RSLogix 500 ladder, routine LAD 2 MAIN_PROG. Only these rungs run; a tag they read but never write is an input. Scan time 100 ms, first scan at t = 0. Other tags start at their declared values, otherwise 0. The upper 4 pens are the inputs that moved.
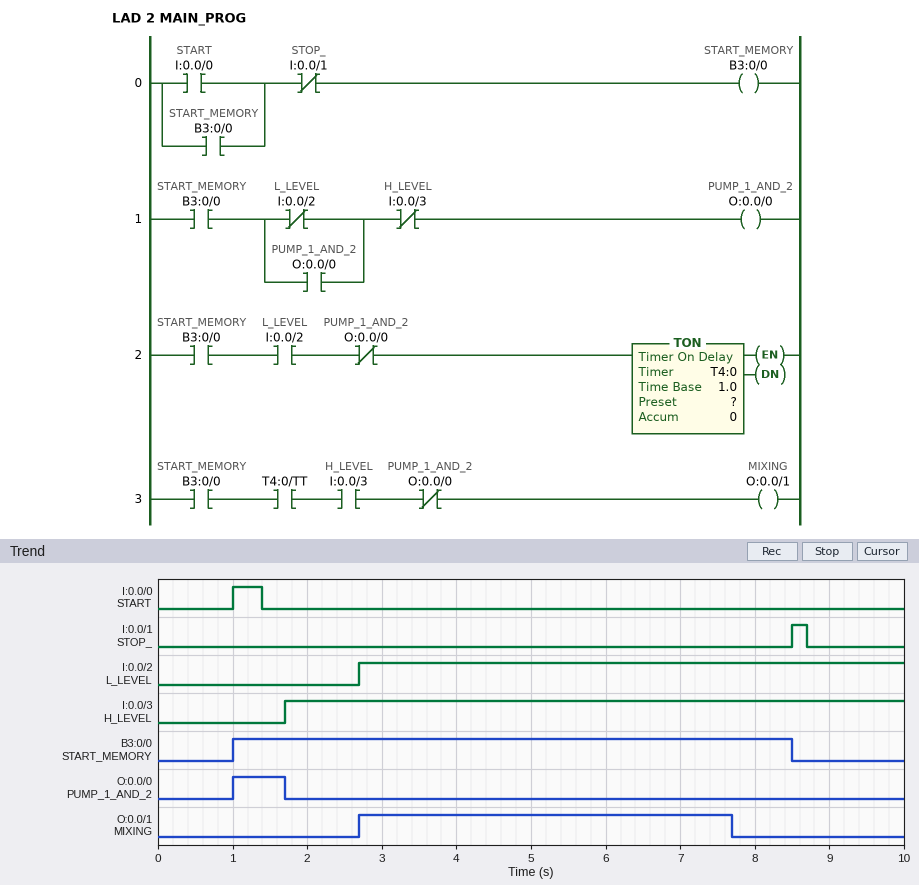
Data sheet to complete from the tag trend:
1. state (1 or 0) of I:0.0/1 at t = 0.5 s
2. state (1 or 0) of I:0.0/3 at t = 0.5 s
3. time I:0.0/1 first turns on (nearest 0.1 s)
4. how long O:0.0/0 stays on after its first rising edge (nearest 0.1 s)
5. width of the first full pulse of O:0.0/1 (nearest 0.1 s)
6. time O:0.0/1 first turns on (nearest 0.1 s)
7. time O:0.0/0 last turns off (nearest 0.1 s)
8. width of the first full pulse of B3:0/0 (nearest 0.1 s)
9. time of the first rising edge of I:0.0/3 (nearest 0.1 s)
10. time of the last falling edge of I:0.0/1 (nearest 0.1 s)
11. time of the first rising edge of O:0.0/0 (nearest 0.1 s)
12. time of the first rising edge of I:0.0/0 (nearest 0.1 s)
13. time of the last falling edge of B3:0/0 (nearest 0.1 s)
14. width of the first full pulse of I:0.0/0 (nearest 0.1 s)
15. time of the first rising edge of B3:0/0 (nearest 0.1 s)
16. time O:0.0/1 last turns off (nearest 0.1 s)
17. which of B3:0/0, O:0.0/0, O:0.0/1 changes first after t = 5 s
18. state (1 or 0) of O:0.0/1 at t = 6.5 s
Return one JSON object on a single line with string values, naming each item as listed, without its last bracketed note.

{"state (1 or 0) of I:0.0/1 at t = 0.5 s": "0", "state (1 or 0) of I:0.0/3 at t = 0.5 s": "0", "time I:0.0/1 first turns on": "8.5 s", "how long O:0.0/0 stays on after its first rising edge": "0.7 s", "width of the first full pulse of O:0.0/1": "5.0 s", "time O:0.0/1 first turns on": "2.7 s", "time O:0.0/0 last turns off": "1.7 s", "width of the first full pulse of B3:0/0": "7.5 s", "time of the first rising edge of I:0.0/3": "1.7 s", "time of the last falling edge of I:0.0/1": "8.7 s", "time of the first rising edge of O:0.0/0": "1.0 s", "time of the first rising edge of I:0.0/0": "1.0 s", "time of the last falling edge of B3:0/0": "8.5 s", "width of the first full pulse of I:0.0/0": "0.4 s", "time of the first rising edge of B3:0/0": "1.0 s", "time O:0.0/1 last turns off": "7.7 s", "which of B3:0/0, O:0.0/0, O:0.0/1 changes first after t = 5 s": "O:0.0/1", "state (1 or 0) of O:0.0/1 at t = 6.5 s": "1"}
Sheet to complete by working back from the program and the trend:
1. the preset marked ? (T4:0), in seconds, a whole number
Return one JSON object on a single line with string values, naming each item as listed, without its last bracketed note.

{"the preset marked ? (T4:0), in seconds, a whole number": "5 s"}
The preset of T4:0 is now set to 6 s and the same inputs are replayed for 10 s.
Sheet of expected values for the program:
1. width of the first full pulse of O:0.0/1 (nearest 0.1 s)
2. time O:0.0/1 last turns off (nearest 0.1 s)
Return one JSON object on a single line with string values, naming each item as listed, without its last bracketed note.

{"width of the first full pulse of O:0.0/1": "5.8 s", "time O:0.0/1 last turns off": "8.5 s"}
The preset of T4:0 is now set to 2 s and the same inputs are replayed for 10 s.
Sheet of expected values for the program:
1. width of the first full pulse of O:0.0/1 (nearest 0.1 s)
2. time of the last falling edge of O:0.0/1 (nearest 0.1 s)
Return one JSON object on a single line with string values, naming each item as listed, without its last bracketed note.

{"width of the first full pulse of O:0.0/1": "2.0 s", "time of the last falling edge of O:0.0/1": "4.7 s"}
